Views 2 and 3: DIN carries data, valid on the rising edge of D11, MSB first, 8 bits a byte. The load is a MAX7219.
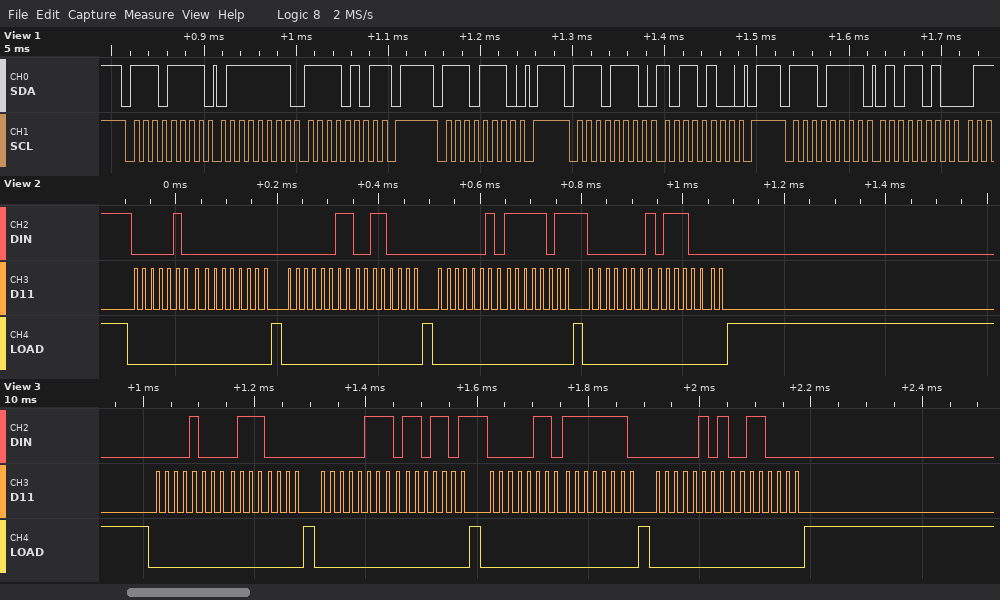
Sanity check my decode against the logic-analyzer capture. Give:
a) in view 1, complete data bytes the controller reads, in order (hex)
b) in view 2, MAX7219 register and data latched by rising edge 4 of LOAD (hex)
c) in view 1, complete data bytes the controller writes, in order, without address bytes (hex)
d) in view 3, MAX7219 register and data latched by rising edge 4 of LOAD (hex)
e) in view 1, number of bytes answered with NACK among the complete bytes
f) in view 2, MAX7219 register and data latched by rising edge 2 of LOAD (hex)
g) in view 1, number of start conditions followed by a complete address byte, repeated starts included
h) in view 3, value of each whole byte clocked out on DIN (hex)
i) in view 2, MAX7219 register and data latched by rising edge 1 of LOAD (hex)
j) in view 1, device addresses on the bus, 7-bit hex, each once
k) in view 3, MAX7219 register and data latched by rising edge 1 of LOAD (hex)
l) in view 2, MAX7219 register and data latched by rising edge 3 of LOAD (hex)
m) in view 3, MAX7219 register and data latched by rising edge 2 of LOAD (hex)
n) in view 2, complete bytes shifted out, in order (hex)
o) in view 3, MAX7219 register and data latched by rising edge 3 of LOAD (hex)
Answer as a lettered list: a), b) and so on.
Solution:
a) 7F F5 5A
b) register 0x1, data 0x70
c) B4
d) register 0x5, data 0x30
e) 1
f) register 0x3, data 0x30
g) 4
h) 08 70 07 6D 06 FE 05 30
i) register 0x4, data 0x00
j) 0x77
k) register 0x8, data 0x70
l) register 0x2, data 0xFB
m) register 0x7, data 0x6D
n) 04 00 03 30 02 FB 01 70
o) register 0x6, data 0xFE
